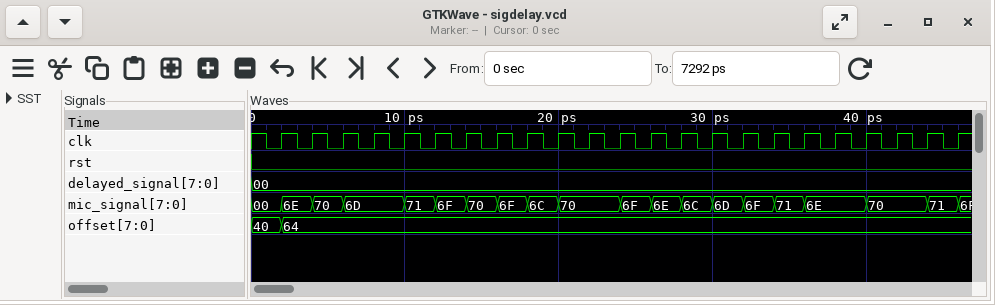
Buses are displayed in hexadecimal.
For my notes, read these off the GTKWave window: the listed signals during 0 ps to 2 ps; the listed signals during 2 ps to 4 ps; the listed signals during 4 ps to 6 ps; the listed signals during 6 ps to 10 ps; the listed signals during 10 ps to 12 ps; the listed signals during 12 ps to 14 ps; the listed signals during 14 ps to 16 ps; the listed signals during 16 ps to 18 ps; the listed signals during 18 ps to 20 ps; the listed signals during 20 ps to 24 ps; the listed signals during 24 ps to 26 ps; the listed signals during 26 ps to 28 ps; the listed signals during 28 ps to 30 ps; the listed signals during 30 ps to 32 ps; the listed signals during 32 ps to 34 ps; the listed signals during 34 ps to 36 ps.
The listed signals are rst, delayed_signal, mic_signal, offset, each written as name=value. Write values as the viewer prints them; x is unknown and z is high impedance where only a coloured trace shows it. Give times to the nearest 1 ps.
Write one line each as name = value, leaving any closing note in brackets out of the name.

the listed signals during 0 ps to 2 ps = rst=0, delayed_signal=00, mic_signal=00, offset=40
the listed signals during 2 ps to 4 ps = rst=0, delayed_signal=00, mic_signal=6E, offset=64
the listed signals during 4 ps to 6 ps = rst=0, delayed_signal=00, mic_signal=70, offset=64
the listed signals during 6 ps to 10 ps = rst=0, delayed_signal=00, mic_signal=6D, offset=64
the listed signals during 10 ps to 12 ps = rst=0, delayed_signal=00, mic_signal=71, offset=64
the listed signals during 12 ps to 14 ps = rst=0, delayed_signal=00, mic_signal=6F, offset=64
the listed signals during 14 ps to 16 ps = rst=0, delayed_signal=00, mic_signal=70, offset=64
the listed signals during 16 ps to 18 ps = rst=0, delayed_signal=00, mic_signal=6F, offset=64
the listed signals during 18 ps to 20 ps = rst=0, delayed_signal=00, mic_signal=6C, offset=64
the listed signals during 20 ps to 24 ps = rst=0, delayed_signal=00, mic_signal=70, offset=64
the listed signals during 24 ps to 26 ps = rst=0, delayed_signal=00, mic_signal=6F, offset=64
the listed signals during 26 ps to 28 ps = rst=0, delayed_signal=00, mic_signal=6E, offset=64
the listed signals during 28 ps to 30 ps = rst=0, delayed_signal=00, mic_signal=6C, offset=64
the listed signals during 30 ps to 32 ps = rst=0, delayed_signal=00, mic_signal=6D, offset=64
the listed signals during 32 ps to 34 ps = rst=0, delayed_signal=00, mic_signal=6F, offset=64
the listed signals during 34 ps to 36 ps = rst=0, delayed_signal=00, mic_signal=71, offset=64
